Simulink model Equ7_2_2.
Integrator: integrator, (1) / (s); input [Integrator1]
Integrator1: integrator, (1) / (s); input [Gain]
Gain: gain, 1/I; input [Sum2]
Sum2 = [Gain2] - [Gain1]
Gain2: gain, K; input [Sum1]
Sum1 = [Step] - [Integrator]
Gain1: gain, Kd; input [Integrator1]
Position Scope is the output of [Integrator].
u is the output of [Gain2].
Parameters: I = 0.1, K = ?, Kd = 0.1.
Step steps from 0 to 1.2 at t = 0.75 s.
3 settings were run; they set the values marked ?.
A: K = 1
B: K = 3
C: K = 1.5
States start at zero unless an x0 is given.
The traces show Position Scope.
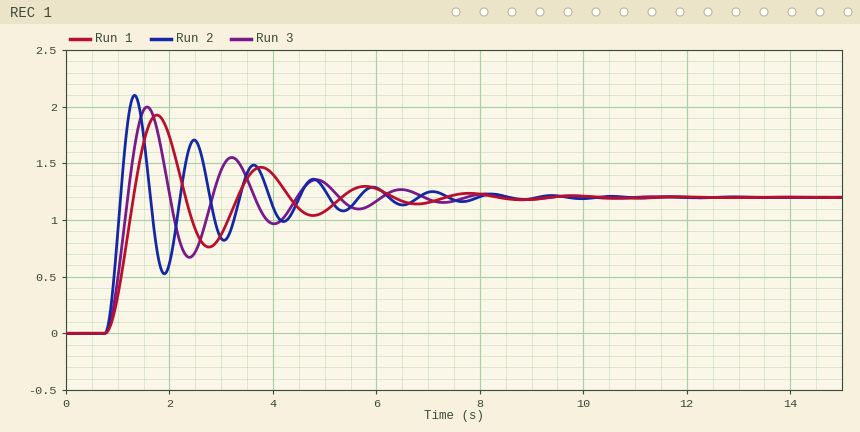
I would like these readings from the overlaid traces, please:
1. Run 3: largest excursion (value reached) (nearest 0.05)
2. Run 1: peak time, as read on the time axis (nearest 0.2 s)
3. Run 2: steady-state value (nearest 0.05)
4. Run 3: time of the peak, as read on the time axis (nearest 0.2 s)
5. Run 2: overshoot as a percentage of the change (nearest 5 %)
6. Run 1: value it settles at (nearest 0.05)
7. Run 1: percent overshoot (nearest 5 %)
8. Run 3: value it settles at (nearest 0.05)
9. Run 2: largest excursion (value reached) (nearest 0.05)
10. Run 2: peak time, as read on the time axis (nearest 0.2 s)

2.00
1.8 s
1.20
1.6 s
75 %
1.20
60 %
1.20
2.10
1.4 s
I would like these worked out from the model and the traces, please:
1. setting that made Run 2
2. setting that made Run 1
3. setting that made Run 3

B
A
C
